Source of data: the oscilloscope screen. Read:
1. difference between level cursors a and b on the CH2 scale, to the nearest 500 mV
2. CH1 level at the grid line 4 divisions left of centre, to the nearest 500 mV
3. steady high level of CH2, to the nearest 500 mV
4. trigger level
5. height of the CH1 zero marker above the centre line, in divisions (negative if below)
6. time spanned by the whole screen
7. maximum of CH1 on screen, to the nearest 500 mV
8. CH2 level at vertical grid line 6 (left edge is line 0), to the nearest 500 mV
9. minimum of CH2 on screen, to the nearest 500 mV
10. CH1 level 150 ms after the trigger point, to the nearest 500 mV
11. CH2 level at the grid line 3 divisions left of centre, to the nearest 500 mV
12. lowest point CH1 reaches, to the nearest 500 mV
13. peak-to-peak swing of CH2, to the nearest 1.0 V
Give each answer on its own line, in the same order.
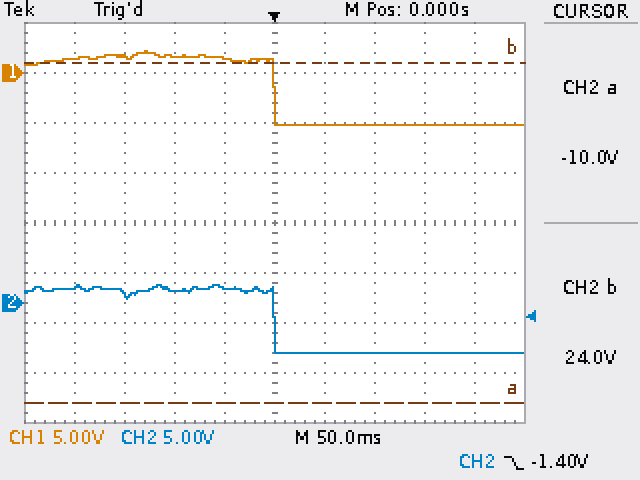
34.0 V
1.5 V
1.5 V
-1.40 V
+3.0 div
500 ms
2.0 V
-5.0 V
-5.0 V
-5.0 V
1.0 V
-5.0 V
7.0 V
